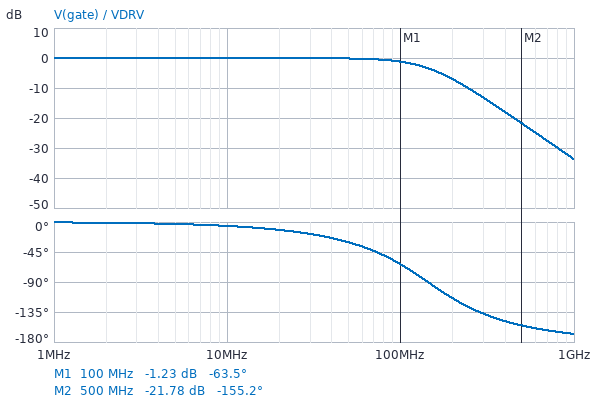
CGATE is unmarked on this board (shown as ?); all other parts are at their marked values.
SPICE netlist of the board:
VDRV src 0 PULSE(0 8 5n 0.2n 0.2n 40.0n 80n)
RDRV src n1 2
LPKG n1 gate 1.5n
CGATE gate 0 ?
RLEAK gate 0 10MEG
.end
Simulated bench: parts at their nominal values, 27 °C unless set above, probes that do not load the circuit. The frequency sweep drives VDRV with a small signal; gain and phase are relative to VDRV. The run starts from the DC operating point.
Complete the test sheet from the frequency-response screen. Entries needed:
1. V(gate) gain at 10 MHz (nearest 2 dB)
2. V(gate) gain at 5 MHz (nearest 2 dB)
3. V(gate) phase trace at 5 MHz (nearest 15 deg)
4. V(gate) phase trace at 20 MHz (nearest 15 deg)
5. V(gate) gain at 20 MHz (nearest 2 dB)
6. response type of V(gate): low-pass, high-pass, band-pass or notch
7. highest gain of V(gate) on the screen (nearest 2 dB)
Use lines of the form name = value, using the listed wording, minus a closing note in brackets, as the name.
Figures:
V(gate) gain at 10 MHz = 0 dB
V(gate) gain at 5 MHz = 0 dB
V(gate) phase trace at 5 MHz = 0 deg
V(gate) phase trace at 20 MHz = -15 deg
V(gate) gain at 20 MHz = 0 dB
response type of V(gate): low-pass, high-pass, band-pass or notch = low-pass
highest gain of V(gate) on the screen = 0 dB
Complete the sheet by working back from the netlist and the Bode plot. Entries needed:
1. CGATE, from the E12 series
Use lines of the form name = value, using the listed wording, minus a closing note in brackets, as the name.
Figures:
CGATE, from the E12 series = 820 pF
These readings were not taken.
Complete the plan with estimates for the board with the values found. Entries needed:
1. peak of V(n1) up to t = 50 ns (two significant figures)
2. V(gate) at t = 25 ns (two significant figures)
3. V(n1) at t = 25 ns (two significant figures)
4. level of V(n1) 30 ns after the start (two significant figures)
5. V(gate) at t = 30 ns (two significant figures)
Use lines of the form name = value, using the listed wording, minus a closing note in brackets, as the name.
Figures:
peak of V(n1) up to t = 50 ns = 8.2 V
V(gate) at t = 25 ns = 8.0 V
V(n1) at t = 25 ns = 8.0 V
level of V(n1) 30 ns after the start = 8.0 V
V(gate) at t = 30 ns = 8.0 V
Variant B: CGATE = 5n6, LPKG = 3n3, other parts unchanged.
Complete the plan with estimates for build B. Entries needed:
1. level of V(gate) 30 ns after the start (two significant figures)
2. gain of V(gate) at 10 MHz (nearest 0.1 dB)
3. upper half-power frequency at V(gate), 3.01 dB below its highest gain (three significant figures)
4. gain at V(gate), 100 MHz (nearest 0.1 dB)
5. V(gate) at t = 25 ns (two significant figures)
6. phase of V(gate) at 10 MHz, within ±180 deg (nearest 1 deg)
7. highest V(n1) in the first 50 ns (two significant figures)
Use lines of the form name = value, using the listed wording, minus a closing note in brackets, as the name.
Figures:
level of V(gate) 30 ns after the start = 7.3 V
gain of V(gate) at 10 MHz = -1.3 dB
upper half-power frequency at V(gate), 3.01 dB below its highest gain = 16.6 MHz
gain at V(gate), 100 MHz = -19.5 dB
V(gate) at t = 25 ns = 6.8 V
phase of V(gate) at 10 MHz, within ±180 deg = -37 deg
highest V(n1) in the first 50 ns = 7.8 V
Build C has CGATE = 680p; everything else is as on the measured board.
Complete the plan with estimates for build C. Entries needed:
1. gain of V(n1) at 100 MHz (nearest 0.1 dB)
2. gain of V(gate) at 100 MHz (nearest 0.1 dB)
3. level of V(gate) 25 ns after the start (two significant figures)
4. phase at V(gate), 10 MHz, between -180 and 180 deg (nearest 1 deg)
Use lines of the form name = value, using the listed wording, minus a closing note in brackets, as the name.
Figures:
gain of V(n1) at 100 MHz = -4.8 dB
gain of V(gate) at 100 MHz = -0.4 dB
level of V(gate) 25 ns after the start = 8.0 V
phase at V(gate), 10 MHz, between -180 and 180 deg = -5 deg
